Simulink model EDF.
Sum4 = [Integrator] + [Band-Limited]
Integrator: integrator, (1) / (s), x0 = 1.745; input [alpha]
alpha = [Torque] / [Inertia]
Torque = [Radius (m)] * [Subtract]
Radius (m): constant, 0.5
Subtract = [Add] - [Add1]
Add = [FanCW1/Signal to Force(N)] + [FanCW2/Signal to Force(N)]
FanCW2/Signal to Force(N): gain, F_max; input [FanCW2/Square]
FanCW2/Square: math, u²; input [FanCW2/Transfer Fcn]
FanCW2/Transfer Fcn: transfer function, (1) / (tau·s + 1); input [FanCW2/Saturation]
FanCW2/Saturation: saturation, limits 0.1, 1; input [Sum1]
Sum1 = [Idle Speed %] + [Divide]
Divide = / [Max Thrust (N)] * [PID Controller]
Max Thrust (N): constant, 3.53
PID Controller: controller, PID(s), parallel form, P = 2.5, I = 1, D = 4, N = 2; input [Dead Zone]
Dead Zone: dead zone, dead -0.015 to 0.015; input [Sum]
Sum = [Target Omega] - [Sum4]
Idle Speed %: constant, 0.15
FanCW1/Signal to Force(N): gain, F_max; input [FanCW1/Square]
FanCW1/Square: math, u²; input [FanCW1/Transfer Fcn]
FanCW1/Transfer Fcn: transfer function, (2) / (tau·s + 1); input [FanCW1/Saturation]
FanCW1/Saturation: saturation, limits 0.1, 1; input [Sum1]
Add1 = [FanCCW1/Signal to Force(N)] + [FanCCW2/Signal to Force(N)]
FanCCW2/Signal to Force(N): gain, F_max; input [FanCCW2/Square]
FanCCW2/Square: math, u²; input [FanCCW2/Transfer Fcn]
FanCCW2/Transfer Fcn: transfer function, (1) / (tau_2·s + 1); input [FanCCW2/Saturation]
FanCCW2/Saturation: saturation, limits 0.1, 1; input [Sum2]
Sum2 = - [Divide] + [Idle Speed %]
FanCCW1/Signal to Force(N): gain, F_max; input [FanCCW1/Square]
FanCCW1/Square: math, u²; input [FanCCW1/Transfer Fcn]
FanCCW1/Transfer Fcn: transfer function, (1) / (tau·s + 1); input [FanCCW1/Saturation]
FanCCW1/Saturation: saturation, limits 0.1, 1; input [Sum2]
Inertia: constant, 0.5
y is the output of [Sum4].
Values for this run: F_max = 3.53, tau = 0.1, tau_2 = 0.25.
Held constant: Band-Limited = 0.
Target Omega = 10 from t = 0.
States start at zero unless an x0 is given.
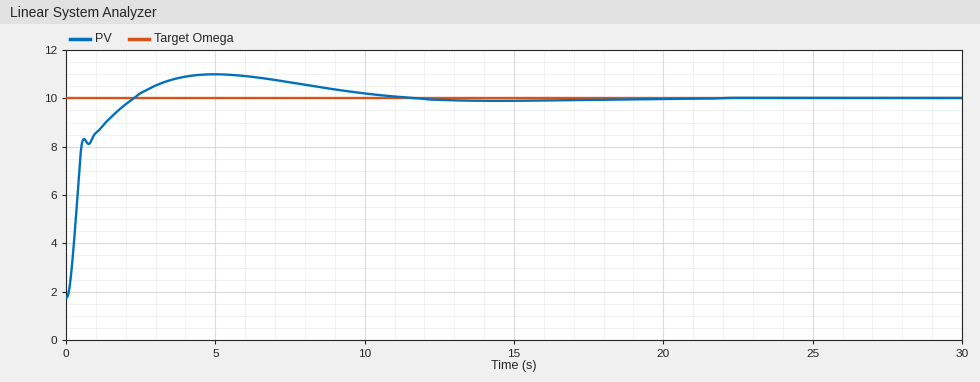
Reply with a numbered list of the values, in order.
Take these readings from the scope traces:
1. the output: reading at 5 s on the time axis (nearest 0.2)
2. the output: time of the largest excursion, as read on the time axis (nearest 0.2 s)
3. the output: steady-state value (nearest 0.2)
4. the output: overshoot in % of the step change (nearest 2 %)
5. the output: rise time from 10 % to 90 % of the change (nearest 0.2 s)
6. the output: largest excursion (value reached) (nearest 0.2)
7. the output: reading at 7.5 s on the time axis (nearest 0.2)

1. 11.0
2. 5.0 s
3. 10.0
4. 12 %
5. 1.4 s
6. 11.0
7. 10.6
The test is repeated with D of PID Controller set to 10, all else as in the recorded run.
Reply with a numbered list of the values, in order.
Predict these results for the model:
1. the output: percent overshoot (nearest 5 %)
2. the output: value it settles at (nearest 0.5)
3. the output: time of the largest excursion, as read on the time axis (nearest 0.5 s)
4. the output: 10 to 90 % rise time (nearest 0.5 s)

1. 15 %
2. 10.0
3. 8.0 s
4. 2.5 s
